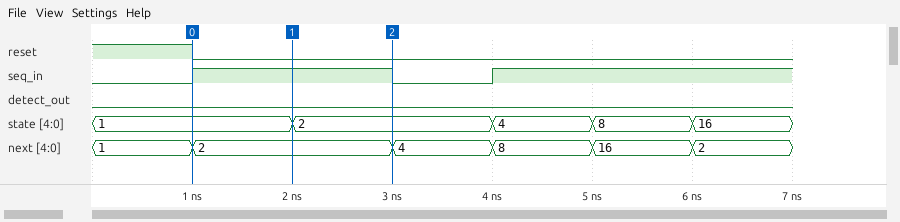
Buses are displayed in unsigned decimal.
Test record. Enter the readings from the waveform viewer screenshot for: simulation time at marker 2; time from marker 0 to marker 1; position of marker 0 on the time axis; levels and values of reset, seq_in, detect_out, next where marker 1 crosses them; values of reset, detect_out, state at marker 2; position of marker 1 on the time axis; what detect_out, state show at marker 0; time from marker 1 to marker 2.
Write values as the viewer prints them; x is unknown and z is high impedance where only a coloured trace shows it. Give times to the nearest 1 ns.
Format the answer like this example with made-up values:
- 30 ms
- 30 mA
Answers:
- 3 ns
- 1 ns
- 1 ns
- reset=0, seq_in=1, detect_out=0, next=2
- reset=0, detect_out=0, state=2
- 2 ns
- detect_out=0, state=1
- 1 ns
